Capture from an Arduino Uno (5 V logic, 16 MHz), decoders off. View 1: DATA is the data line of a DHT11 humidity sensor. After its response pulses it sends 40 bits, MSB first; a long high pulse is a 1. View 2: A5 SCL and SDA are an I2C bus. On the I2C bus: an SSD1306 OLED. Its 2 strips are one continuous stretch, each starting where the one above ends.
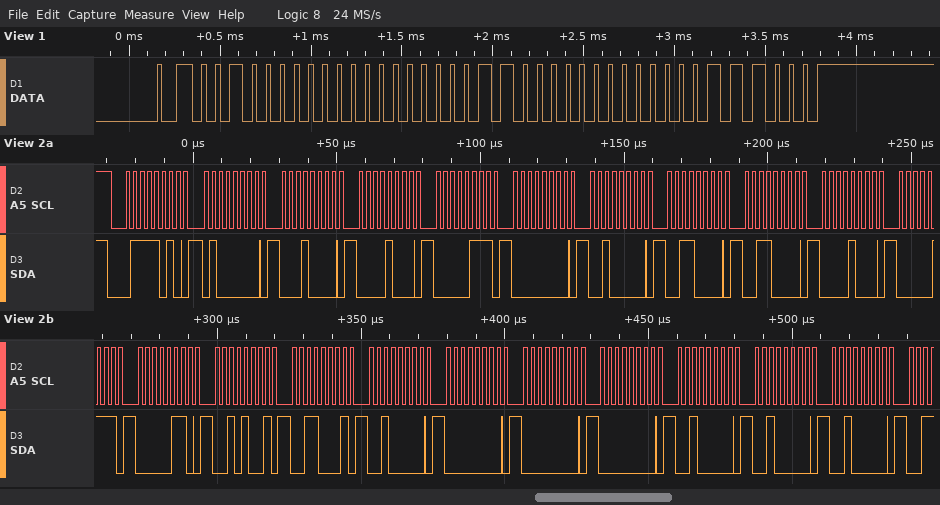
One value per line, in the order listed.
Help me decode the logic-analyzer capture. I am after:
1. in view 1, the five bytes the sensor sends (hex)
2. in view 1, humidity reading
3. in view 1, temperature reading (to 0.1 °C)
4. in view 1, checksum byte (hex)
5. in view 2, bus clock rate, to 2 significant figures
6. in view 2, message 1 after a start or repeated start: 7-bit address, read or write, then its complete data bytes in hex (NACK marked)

20 00 18 00 38
32 %
24.0 °C
0x38
400 kHz
0x3D write: 40 10 08 07 00 20 30 30 08 07 06 29 31 20 00 00 00 20 20 20
